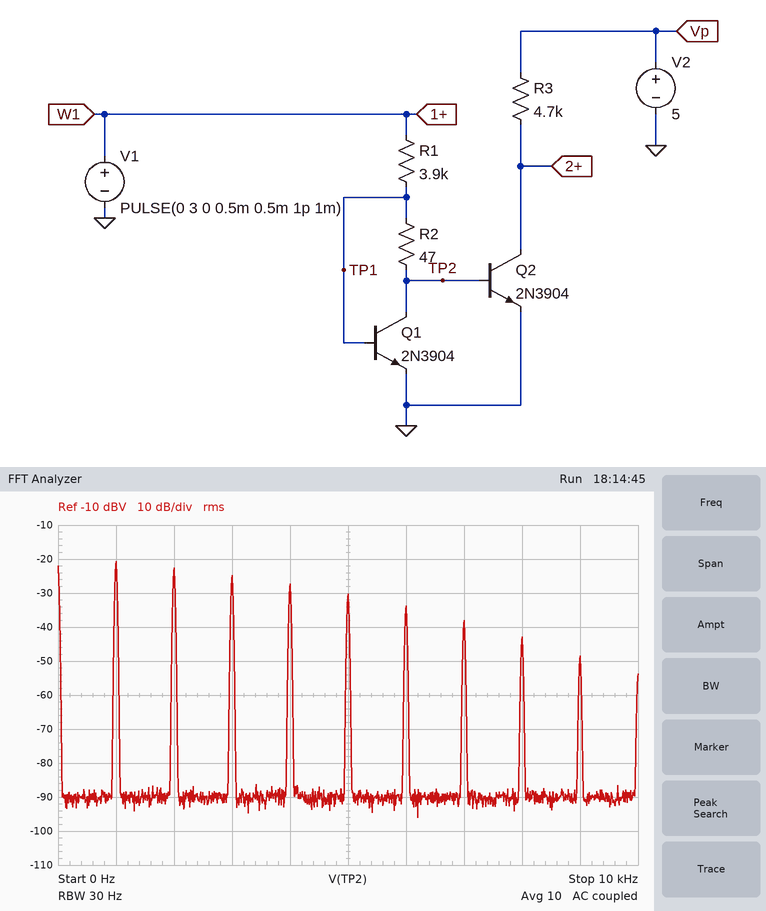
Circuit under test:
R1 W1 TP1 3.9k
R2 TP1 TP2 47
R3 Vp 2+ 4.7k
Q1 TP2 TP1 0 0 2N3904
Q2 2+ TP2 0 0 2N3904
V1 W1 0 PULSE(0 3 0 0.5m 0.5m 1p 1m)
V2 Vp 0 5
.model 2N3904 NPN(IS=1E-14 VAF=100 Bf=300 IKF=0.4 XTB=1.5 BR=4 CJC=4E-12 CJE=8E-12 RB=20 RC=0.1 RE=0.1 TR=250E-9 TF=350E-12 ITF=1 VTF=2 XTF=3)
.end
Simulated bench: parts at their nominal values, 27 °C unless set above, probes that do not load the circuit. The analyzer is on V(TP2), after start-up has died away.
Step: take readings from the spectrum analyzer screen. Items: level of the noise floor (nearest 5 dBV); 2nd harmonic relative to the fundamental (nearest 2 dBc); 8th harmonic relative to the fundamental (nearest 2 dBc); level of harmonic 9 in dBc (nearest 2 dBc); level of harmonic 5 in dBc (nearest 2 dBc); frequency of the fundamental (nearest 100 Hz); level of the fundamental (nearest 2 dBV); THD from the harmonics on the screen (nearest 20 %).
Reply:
-90 dBV
-2 dBc
-22 dBc
-28 dBc
-10 dBc
1.0 kHz
-20 dBV
120 %
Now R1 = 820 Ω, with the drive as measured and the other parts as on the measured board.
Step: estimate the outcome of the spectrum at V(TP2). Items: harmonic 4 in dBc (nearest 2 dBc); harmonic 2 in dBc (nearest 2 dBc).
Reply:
-4 dBc
2 dBc
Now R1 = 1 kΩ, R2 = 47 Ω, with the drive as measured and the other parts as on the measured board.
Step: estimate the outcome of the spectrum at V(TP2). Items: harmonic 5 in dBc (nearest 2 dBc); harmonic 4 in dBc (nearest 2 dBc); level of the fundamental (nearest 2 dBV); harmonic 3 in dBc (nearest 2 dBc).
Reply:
-8 dBc
-4 dBc
-22 dBV
-2 dBc
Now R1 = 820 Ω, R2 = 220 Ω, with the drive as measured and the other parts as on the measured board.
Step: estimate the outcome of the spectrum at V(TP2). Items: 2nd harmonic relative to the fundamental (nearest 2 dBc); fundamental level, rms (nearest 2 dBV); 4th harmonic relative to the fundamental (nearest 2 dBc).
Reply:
2 dBc
-22 dBV
-4 dBc
